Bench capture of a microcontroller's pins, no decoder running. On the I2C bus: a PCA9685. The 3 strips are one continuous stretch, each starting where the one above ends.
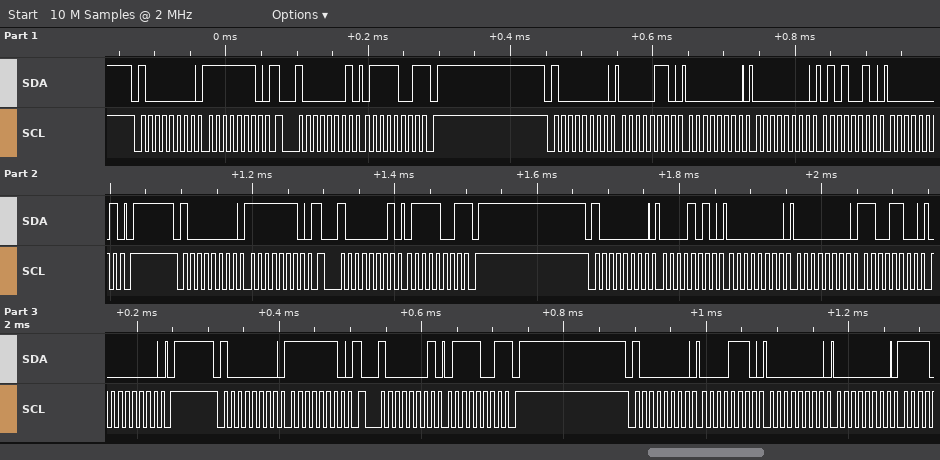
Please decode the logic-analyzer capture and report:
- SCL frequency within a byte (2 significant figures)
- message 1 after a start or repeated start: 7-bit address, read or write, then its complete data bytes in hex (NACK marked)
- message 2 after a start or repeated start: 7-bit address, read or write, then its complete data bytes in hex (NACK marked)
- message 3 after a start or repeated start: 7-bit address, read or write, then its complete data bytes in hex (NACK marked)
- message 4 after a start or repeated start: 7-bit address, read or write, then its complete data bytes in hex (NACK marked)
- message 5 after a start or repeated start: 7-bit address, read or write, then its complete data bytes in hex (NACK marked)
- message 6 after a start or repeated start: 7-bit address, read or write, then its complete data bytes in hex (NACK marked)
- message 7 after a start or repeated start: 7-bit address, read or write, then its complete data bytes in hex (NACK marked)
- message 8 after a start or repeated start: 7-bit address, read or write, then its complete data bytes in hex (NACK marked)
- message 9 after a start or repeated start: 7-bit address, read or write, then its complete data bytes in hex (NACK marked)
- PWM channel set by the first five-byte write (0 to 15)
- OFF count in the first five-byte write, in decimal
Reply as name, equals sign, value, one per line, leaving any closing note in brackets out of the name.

SCL frequency within a byte = 100 kHz
message 1 after a start or repeated start: 7-bit address, read or write, then its complete data bytes in hex = 0x40 write: FE
message 2 after a start or repeated start: 7-bit address, read or write, then its complete data bytes in hex = 0x40 read: 79 NACK
message 3 after a start or repeated start: 7-bit address, read or write, then its complete data bytes in hex = 0x40 write: 06 00 00 52 01
message 4 after a start or repeated start: 7-bit address, read or write, then its complete data bytes in hex = 0x40 write: FE
message 5 after a start or repeated start: 7-bit address, read or write, then its complete data bytes in hex = 0x40 read: 79 NACK
message 6 after a start or repeated start: 7-bit address, read or write, then its complete data bytes in hex = 0x40 write: 0A 00 00 CC 00
message 7 after a start or repeated start: 7-bit address, read or write, then its complete data bytes in hex = 0x40 write: FE
message 8 after a start or repeated start: 7-bit address, read or write, then its complete data bytes in hex = 0x40 read: 79 NACK
message 9 after a start or repeated start: 7-bit address, read or write, then its complete data bytes in hex = 0x40 write: 0E 00 00
PWM channel set by the first five-byte write = 0
OFF count in the first five-byte write, in decimal = 338
